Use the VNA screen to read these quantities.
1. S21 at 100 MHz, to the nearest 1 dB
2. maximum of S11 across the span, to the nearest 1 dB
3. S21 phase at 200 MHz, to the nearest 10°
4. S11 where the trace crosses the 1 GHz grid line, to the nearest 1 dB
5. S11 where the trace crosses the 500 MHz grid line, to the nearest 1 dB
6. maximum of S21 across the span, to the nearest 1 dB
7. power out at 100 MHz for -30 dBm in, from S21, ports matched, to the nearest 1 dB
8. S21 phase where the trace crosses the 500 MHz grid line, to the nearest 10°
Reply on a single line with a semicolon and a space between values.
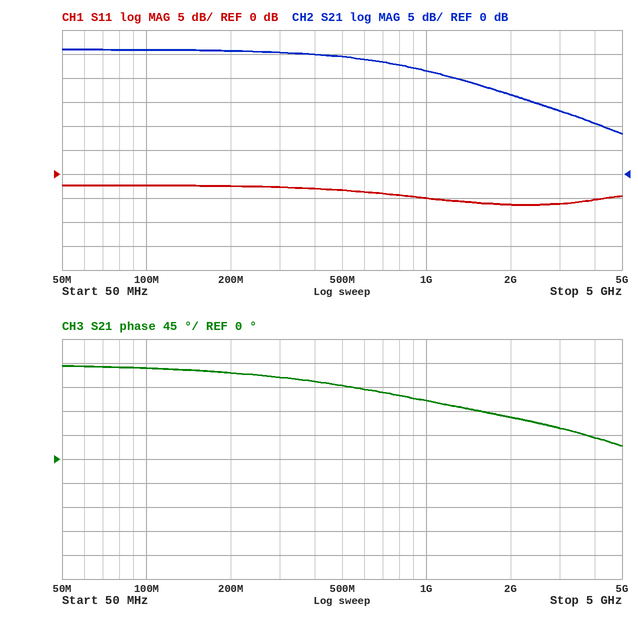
26 dB; -2 dB; 160°; -5 dB; -3 dB; 26 dB; -4 dBm; 140°
